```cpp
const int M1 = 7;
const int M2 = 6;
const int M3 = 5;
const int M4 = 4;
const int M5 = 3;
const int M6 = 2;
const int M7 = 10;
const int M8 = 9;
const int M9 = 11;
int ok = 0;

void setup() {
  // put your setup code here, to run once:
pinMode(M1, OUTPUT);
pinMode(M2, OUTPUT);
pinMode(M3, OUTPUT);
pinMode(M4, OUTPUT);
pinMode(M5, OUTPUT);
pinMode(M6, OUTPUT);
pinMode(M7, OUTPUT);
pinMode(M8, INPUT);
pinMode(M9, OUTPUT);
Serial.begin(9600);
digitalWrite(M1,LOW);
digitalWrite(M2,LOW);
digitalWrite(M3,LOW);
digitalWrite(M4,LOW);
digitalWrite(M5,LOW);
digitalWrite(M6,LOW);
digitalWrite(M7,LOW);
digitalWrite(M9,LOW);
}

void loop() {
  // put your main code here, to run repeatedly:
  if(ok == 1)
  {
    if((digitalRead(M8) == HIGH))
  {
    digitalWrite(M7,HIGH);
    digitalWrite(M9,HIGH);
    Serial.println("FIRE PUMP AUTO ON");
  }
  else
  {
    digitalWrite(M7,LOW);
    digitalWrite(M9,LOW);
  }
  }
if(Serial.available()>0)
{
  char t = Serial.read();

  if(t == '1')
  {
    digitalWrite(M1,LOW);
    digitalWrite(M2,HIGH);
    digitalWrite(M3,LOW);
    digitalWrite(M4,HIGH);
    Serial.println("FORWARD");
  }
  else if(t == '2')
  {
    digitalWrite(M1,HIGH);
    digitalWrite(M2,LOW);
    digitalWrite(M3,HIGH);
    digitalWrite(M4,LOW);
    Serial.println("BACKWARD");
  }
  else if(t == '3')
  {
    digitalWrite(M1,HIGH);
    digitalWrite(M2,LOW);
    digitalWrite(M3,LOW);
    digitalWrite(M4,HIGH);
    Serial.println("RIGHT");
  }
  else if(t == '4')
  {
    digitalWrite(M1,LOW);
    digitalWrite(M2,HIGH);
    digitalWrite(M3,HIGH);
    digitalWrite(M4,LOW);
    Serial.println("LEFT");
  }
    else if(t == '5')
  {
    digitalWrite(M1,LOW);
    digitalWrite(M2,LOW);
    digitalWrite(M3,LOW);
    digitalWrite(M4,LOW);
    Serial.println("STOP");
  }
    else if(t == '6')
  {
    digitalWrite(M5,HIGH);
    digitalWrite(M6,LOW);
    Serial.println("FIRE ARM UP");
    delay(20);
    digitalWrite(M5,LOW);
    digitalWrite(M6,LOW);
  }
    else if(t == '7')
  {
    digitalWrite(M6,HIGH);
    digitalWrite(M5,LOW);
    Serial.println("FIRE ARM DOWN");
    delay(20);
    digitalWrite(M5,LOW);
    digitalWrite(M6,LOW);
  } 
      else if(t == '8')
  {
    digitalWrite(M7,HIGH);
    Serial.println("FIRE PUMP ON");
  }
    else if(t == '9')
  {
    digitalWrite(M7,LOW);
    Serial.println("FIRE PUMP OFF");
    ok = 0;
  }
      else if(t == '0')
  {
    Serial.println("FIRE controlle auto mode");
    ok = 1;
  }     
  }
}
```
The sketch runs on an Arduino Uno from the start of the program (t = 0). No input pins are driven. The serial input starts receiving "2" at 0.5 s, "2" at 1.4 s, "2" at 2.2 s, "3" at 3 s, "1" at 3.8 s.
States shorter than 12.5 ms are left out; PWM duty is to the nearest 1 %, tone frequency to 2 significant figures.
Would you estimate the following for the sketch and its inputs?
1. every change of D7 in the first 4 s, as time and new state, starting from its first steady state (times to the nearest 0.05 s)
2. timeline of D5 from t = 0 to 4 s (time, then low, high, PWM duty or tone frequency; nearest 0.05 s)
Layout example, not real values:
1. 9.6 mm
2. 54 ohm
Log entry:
1. 0 s low; 0.5 s high; 3.8 s low
2. 0 s low; 0.5 s high; 3 s low
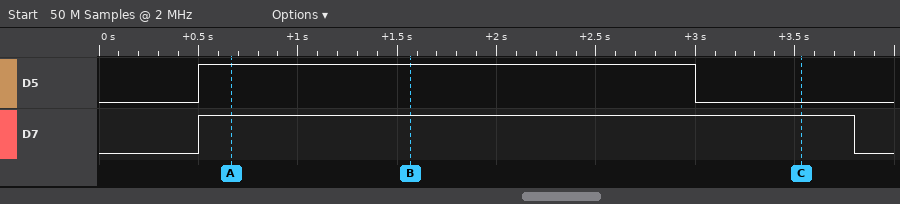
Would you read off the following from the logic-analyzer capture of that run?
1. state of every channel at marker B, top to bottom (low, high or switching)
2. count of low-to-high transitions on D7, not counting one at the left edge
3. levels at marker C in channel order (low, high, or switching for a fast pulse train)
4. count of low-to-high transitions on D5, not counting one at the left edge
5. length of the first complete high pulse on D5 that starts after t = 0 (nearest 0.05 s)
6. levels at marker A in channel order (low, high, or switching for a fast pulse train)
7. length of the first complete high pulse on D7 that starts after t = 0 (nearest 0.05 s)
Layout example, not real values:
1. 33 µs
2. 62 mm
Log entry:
1. D5 high, D7 high
2. 1
3. D5 low, D7 high
4. 1
5. 2.50 s
6. D5 high, D7 high
7. 3.30 s
